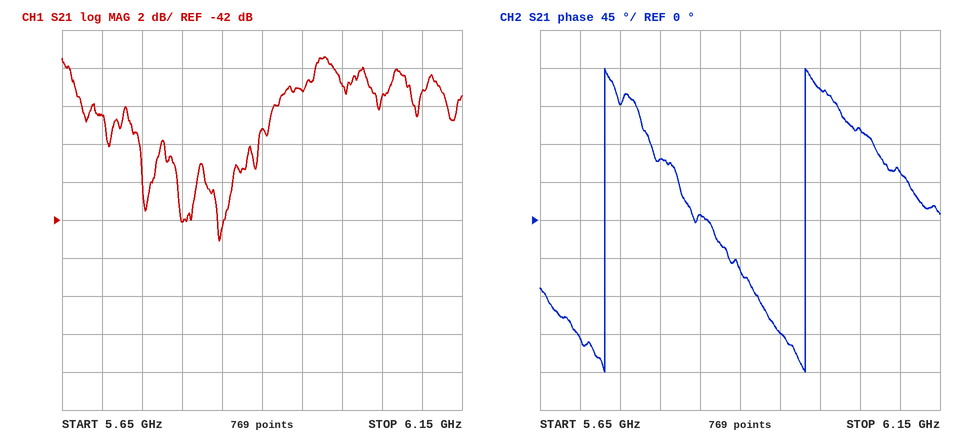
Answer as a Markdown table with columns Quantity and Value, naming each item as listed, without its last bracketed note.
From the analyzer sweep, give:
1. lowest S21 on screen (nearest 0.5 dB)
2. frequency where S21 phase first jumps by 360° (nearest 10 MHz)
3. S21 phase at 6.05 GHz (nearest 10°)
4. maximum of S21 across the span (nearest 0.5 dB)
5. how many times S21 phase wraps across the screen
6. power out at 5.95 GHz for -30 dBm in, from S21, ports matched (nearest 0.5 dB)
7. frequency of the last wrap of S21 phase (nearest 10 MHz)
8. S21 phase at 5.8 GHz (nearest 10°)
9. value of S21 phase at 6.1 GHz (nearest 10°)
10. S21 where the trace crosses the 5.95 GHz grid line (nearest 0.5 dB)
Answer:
| Quantity | Value |
|---|---|
| lowest S21 on screen | -43.0 dB |
| frequency where S21 phase first jumps by 360° | 5.73 GHz |
| S21 phase at 6.05 GHz | 110° |
| maximum of S21 across the span | -33.5 dB |
| how many times S21 phase wraps across the screen | 2 |
| power out at 5.95 GHz for -30 dBm in, from S21, ports matched | -65.0 dBm |
| frequency of the last wrap of S21 phase | 5.98 GHz |
| S21 phase at 5.8 GHz | 70° |
| value of S21 phase at 6.1 GHz | 60° |
| S21 where the trace crosses the 5.95 GHz grid line | -35.0 dB |
